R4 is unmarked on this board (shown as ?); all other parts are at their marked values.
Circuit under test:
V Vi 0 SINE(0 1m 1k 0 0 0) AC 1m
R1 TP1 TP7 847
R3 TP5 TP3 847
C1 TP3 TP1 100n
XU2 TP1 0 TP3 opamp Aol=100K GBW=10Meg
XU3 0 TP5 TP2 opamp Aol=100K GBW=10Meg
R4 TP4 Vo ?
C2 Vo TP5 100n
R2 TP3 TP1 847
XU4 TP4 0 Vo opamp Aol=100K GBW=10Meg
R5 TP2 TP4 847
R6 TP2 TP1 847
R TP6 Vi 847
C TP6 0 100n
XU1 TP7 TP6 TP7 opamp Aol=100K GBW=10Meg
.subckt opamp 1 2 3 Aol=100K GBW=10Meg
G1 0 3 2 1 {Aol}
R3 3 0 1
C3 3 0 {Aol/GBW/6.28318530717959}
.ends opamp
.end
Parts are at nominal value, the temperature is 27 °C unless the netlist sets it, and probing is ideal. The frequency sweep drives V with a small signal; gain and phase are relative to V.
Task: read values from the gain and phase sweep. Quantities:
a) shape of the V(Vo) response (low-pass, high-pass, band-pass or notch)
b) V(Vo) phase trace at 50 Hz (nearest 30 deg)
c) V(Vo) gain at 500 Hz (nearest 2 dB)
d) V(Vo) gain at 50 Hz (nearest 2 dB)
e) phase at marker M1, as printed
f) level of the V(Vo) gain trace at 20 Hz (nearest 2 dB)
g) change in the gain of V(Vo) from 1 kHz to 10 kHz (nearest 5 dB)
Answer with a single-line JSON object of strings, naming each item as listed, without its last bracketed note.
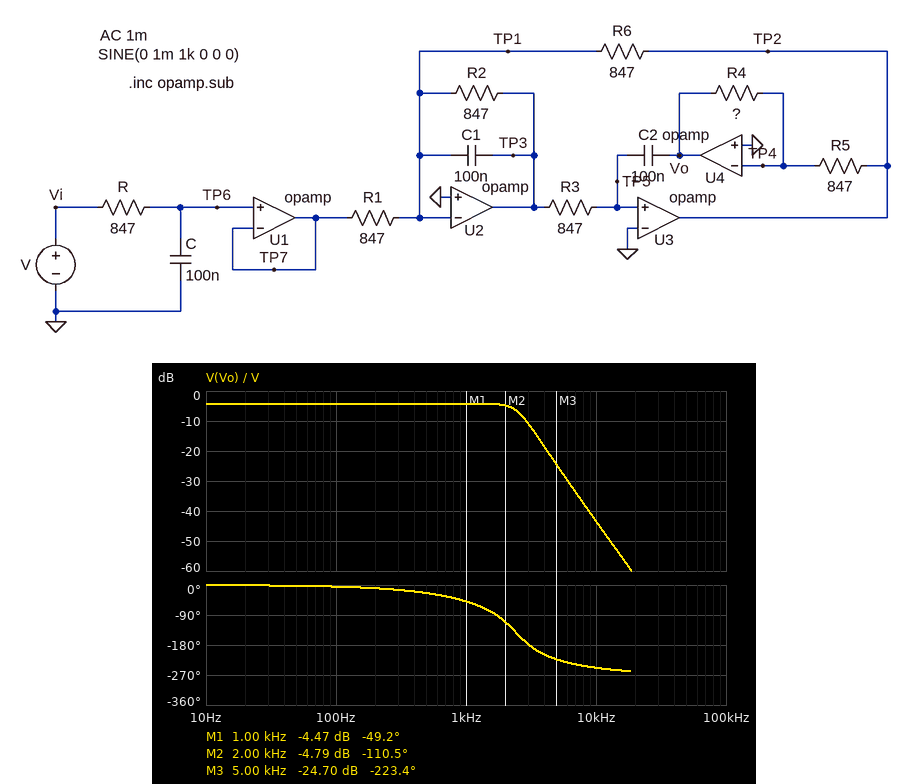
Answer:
{"shape of the V(Vo) response": "low-pass", "V(Vo) phase trace at 50 Hz": "0 deg", "V(Vo) gain at 500 Hz": "-4 dB", "V(Vo) gain at 50 Hz": "-4 dB", "phase at marker M1, as printed": "-49.2 deg", "level of the V(Vo) gain trace at 20 Hz": "-4 dB", "change in the gain of V(Vo) from 1 kHz to 10 kHz": "-40 dB"}
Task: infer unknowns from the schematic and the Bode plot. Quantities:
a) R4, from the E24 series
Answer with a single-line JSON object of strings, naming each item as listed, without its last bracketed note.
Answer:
{"R4, from the E24 series": "510 Ω"}
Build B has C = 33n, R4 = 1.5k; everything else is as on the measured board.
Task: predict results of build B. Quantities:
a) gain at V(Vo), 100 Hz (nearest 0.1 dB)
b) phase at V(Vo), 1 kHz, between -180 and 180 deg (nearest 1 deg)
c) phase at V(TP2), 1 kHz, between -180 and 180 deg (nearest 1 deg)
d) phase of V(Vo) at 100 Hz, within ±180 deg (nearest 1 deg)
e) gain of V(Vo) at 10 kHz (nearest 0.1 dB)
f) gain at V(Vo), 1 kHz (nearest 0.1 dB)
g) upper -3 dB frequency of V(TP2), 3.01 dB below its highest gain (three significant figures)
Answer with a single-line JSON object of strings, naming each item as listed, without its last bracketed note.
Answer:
{"gain at V(Vo), 100 Hz": "5.0 dB", "phase at V(Vo), 1 kHz, between -180 and 180 deg": "-72 deg", "phase at V(TP2), 1 kHz, between -180 and 180 deg": "108 deg", "phase of V(Vo) at 100 Hz, within ±180 deg": "-6 deg", "gain of V(Vo) at 10 kHz": "-35.1 dB", "gain at V(Vo), 1 kHz": "4.3 dB", "upper -3 dB frequency of V(TP2), 3.01 dB below its highest gain": "1.45 kHz"}
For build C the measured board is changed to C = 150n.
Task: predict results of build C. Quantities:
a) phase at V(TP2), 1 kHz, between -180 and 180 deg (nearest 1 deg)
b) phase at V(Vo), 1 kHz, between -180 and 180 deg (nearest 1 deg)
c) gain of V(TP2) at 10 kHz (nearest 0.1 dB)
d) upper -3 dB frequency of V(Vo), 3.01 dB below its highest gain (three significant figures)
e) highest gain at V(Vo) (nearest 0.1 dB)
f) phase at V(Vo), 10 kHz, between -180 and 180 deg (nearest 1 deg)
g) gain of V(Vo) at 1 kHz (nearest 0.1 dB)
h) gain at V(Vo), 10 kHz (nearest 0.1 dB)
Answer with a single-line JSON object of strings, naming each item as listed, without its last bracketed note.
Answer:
{"phase at V(TP2), 1 kHz, between -180 and 180 deg": "120 deg", "phase at V(Vo), 1 kHz, between -180 and 180 deg": "-60 deg", "gain of V(TP2) at 10 kHz": "-42.4 dB", "upper -3 dB frequency of V(Vo), 3.01 dB below its highest gain": "2.12 kHz", "highest gain at V(Vo)": "-4.4 dB", "phase at V(Vo), 10 kHz, between -180 and 180 deg": "108 deg", "gain of V(Vo) at 1 kHz": "-5.5 dB", "gain at V(Vo), 10 kHz": "-46.8 dB"}
